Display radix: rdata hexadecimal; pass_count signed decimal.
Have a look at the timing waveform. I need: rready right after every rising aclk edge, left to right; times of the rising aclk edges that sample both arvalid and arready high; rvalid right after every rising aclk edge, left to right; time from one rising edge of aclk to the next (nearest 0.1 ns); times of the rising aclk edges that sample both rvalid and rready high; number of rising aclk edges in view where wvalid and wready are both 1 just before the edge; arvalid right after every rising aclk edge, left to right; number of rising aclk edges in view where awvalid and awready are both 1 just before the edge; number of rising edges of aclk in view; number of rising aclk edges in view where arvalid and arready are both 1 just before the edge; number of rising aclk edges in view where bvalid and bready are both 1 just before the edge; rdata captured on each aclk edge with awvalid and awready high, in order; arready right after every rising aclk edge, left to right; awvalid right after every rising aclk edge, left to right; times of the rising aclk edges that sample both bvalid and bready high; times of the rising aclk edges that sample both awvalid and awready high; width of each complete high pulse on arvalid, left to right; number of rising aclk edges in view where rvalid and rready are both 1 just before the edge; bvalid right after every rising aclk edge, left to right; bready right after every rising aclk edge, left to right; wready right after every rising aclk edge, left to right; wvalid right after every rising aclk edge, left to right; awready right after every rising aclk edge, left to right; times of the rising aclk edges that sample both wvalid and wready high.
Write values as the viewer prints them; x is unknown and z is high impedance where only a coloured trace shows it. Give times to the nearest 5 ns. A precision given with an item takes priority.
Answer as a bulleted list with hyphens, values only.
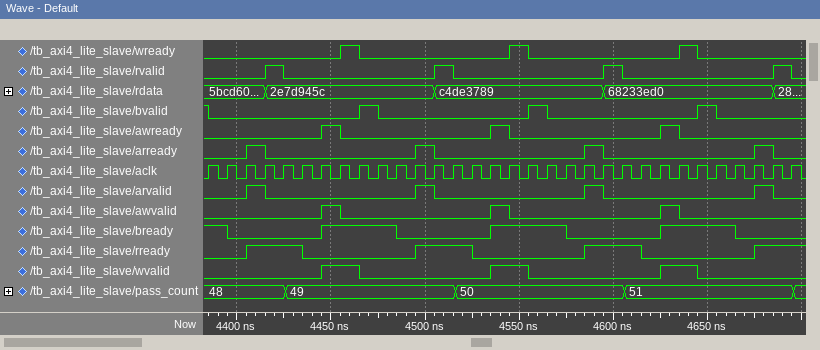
- 0 0 1 1 1 0 0 0 0 0 0 1 1 1 0 0 0 0 0 0 1 1 1 0 0 0 0 0 0 1 1 1
- 4415 ns, 4505 ns, 4595 ns, 4685 ns
- 0 0 0 1 0 0 0 0 0 0 0 0 1 0 0 0 0 0 0 0 0 1 0 0 0 0 0 0 0 0 1 0
- 10 ns
- 4425 ns, 4515 ns, 4605 ns, 4695 ns
- 3
- 0 0 1 0 0 0 0 0 0 0 0 1 0 0 0 0 0 0 0 0 1 0 0 0 0 0 0 0 0 1 0 0
- 3
- 32
- 4
- 4
- 2e7d945c, c4de3789, 68233ed0
- 0 0 1 0 0 0 0 0 0 0 0 1 0 0 0 0 0 0 0 0 1 0 0 0 0 0 0 0 0 1 0 0
- 0 0 0 0 0 0 1 0 0 0 0 0 0 0 0 1 0 0 0 0 0 0 0 0 1 0 0 0 0 0 0 0
- 4385 ns, 4475 ns, 4565 ns, 4655 ns
- 4455 ns, 4545 ns, 4635 ns
- 10 ns, 10 ns, 10 ns, 10 ns
- 4
- 0 0 0 0 0 0 0 0 1 0 0 0 0 0 0 0 0 1 0 0 0 0 0 0 0 0 1 0 0 0 0 0
- 1 0 0 0 0 0 1 1 1 1 0 0 0 0 0 1 1 1 1 0 0 0 0 0 1 1 1 1 0 0 0 0
- 0 0 0 0 0 0 0 1 0 0 0 0 0 0 0 0 1 0 0 0 0 0 0 0 0 1 0 0 0 0 0 0
- 0 0 0 0 0 0 1 1 0 0 0 0 0 0 0 1 1 0 0 0 0 0 0 0 1 1 0 0 0 0 0 0
- 0 0 0 0 0 0 1 0 0 0 0 0 0 0 0 1 0 0 0 0 0 0 0 0 1 0 0 0 0 0 0 0
- 4465 ns, 4555 ns, 4645 ns
